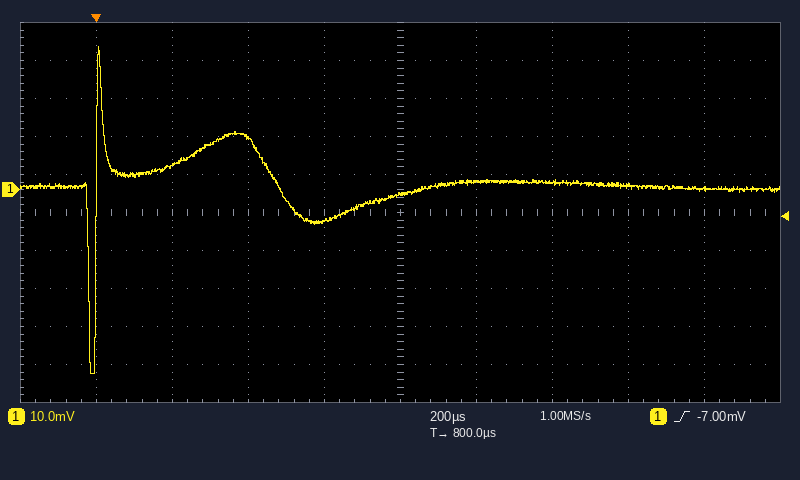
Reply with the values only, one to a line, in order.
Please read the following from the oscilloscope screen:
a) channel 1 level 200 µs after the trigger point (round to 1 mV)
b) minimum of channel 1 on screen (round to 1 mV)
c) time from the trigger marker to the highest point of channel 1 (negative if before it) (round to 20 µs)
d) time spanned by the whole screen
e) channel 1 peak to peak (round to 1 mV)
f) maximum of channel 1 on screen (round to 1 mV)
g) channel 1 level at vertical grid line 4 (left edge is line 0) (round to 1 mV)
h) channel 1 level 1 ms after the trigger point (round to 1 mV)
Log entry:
6 mV
-48 mV
0 µs
2 ms
86 mV
38 mV
-8 mV
2 mV
